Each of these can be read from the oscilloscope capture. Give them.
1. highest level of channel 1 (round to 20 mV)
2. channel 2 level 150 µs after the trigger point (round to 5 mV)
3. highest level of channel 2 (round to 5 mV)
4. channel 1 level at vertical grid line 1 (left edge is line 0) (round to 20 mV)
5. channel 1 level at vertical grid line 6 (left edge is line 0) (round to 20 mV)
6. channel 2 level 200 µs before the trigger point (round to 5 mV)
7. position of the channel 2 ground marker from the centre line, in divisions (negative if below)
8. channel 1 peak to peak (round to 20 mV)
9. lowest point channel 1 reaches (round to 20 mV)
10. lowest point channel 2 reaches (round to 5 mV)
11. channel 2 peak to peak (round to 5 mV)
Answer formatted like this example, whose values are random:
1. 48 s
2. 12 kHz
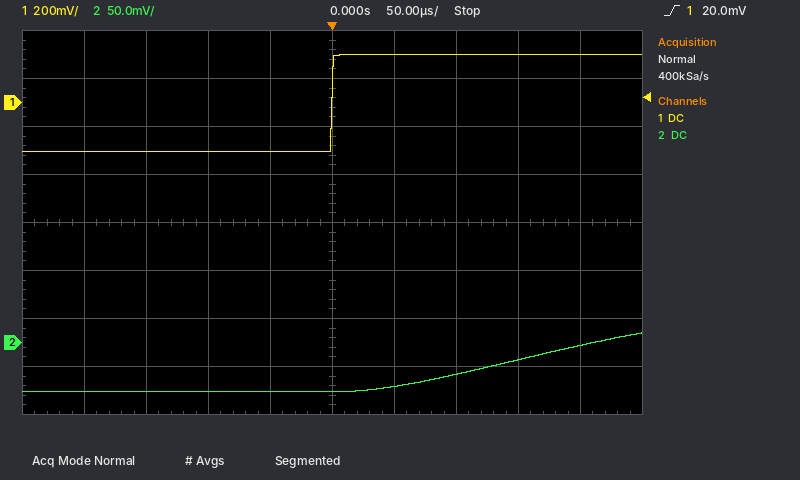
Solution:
1. 200 mV
2. -20 mV
3. 10 mV
4. -200 mV
5. 200 mV
6. -50 mV
7. -2.5 div
8. 400 mV
9. -200 mV
10. -50 mV
11. 60 mV
